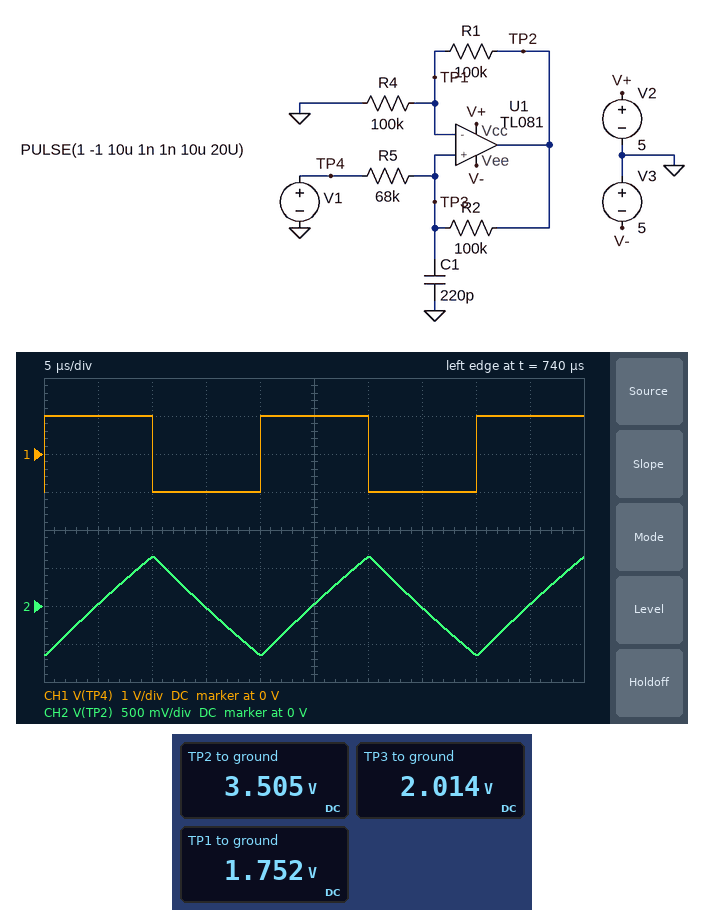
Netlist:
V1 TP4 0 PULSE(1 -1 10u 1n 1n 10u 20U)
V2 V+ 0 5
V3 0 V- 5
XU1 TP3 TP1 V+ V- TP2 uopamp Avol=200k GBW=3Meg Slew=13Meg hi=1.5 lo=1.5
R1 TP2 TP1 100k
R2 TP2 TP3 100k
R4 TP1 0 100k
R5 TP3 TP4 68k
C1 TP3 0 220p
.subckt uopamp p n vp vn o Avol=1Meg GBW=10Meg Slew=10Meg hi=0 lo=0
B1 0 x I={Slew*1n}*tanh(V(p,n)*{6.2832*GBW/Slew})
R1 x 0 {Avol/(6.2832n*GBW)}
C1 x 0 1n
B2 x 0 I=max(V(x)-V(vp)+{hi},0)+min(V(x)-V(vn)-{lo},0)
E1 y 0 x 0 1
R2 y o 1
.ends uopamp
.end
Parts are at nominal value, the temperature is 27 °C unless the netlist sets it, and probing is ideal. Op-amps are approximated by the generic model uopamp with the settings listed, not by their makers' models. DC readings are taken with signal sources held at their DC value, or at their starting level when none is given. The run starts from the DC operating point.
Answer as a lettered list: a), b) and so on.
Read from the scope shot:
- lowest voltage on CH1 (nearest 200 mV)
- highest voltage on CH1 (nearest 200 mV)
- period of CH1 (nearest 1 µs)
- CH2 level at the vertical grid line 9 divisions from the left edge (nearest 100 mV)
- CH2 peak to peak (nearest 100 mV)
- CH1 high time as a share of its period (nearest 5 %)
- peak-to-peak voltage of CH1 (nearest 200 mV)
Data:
a) -1.0 V
b) 1.0 V
c) 20 µs
d) 0 V
e) 1.3 V
f) 50 %
g) 2.0 V
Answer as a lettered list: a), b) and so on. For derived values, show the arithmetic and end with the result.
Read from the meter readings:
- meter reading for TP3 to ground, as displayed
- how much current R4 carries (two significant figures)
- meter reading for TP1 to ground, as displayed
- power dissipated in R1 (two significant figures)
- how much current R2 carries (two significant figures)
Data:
a) 2.014 V
b) (1.752 V) / 100 kΩ = 18 µA
c) 1.752 V
d) (3.505 V - 1.752 V)^2 / 100 kΩ = 31 µW
e) (3.505 V - 2.014 V) / 100 kΩ = 15 µA
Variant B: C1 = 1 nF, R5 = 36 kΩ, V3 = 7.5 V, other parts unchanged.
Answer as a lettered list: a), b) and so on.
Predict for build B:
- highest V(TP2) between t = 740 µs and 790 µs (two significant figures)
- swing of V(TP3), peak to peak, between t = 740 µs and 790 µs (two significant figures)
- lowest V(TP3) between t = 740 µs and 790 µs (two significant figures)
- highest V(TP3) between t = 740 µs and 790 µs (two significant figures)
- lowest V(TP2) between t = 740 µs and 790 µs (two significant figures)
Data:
a) 270 mV
b) 280 mV
c) -140 mV
d) 140 mV
e) -270 mV
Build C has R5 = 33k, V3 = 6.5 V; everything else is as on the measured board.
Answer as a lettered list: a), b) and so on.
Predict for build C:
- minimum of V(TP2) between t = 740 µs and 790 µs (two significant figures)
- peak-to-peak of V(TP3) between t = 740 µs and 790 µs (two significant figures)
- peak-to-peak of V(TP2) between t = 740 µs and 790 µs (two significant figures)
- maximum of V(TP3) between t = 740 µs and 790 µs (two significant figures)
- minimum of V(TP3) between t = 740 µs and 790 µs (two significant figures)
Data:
a) -1.3 V
b) 1.3 V
c) 2.5 V
d) 640 mV
e) -640 mV
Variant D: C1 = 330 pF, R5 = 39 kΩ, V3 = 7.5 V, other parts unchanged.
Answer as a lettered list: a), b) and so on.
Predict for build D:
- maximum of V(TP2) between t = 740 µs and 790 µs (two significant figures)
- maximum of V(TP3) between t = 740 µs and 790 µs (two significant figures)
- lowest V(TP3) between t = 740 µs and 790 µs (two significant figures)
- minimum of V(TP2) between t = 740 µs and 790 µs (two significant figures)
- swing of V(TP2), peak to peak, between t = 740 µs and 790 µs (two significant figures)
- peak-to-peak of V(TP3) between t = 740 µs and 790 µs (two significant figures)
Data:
a) 750 mV
b) 380 mV
c) -380 mV
d) -750 mV
e) 1.5 V
f) 760 mV
